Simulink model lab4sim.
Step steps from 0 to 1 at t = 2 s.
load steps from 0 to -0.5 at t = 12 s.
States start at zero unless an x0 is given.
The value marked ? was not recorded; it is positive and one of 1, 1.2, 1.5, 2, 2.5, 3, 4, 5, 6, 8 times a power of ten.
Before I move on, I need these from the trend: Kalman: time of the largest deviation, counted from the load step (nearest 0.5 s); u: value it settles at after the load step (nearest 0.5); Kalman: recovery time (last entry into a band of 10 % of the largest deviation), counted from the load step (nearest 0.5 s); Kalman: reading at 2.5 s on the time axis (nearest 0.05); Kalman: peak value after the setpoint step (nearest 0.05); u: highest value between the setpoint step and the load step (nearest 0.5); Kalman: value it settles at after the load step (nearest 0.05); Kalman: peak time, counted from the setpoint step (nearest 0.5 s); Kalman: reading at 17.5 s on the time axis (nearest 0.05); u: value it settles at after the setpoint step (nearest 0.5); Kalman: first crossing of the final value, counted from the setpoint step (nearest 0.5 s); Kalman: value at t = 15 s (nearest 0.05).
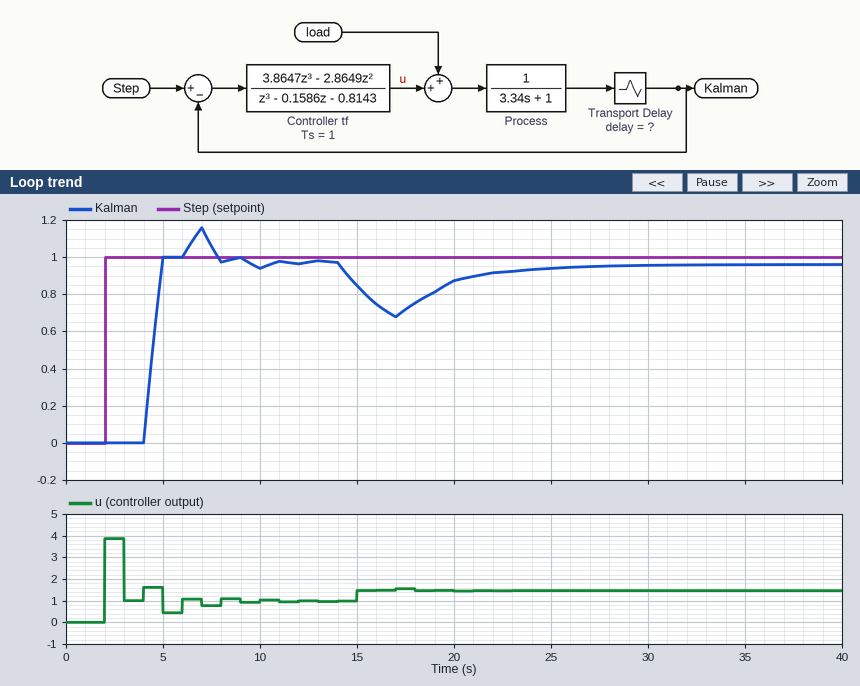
5.0 s
1.5
12.0 s
0.00
1.15
4.0
0.95
5.0 s
0.70
1.0
3.0 s
0.85
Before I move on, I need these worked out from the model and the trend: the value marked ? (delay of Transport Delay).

2
